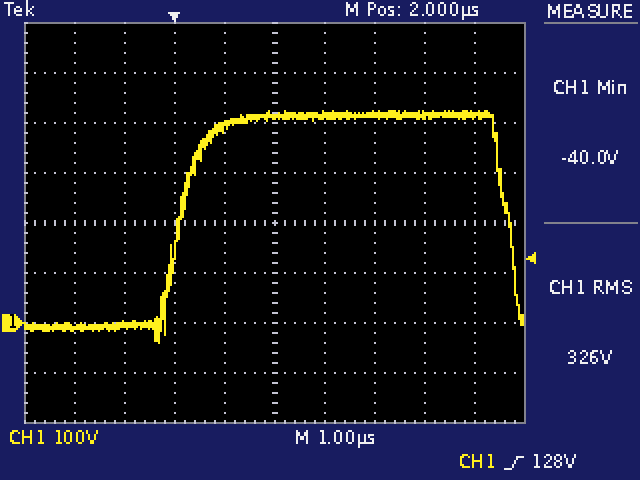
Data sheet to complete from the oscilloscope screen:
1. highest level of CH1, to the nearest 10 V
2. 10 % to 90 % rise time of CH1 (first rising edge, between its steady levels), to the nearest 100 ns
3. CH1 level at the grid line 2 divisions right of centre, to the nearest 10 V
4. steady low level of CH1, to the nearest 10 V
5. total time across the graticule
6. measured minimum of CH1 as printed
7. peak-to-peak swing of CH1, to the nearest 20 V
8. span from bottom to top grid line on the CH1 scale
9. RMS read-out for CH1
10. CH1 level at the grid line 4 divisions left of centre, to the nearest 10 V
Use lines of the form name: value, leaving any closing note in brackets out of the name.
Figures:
highest level of CH1, to the nearest 10 V: 420 V
10 % to 90 % rise time of CH1 (first rising edge, between its steady levels), to the nearest 100 ns: 900 ns
CH1 level at the grid line 2 divisions right of centre, to the nearest 10 V: 420 V
steady low level of CH1, to the nearest 10 V: -10 V
total time across the graticule: 10 µs
measured minimum of CH1 as printed: -40.0 V
peak-to-peak swing of CH1, to the nearest 20 V: 460 V
span from bottom to top grid line on the CH1 scale: 800 V
RMS read-out for CH1: 326 V
CH1 level at the grid line 4 divisions left of centre, to the nearest 10 V: -10 V
